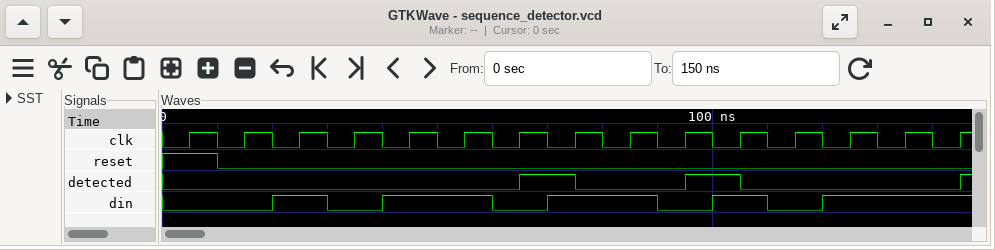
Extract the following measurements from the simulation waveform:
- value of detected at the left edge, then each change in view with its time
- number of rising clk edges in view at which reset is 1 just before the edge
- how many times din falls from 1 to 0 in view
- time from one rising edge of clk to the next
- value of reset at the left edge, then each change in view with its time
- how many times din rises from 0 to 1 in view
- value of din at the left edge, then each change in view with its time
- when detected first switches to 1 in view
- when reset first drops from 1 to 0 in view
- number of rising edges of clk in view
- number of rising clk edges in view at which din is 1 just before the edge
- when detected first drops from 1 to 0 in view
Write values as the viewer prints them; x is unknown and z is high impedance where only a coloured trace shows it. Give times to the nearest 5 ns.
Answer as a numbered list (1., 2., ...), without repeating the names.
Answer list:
1. 0, 1 at 65 ns, 0 at 75 ns, 1 at 95 ns, 0 at 105 ns, 1 at 145 ns
2. 1
3. 4
4. 10 ns
5. 1, 0 at 10 ns
6. 5
7. 0, 1 at 20 ns, 0 at 30 ns, 1 at 40 ns, 0 at 60 ns, 1 at 70 ns, 0 at 90 ns, 1 at 100 ns, 0 at 110 ns, 1 at 120 ns
8. 65 ns
9. 10 ns
10. 15
11. 9
12. 75 ns
